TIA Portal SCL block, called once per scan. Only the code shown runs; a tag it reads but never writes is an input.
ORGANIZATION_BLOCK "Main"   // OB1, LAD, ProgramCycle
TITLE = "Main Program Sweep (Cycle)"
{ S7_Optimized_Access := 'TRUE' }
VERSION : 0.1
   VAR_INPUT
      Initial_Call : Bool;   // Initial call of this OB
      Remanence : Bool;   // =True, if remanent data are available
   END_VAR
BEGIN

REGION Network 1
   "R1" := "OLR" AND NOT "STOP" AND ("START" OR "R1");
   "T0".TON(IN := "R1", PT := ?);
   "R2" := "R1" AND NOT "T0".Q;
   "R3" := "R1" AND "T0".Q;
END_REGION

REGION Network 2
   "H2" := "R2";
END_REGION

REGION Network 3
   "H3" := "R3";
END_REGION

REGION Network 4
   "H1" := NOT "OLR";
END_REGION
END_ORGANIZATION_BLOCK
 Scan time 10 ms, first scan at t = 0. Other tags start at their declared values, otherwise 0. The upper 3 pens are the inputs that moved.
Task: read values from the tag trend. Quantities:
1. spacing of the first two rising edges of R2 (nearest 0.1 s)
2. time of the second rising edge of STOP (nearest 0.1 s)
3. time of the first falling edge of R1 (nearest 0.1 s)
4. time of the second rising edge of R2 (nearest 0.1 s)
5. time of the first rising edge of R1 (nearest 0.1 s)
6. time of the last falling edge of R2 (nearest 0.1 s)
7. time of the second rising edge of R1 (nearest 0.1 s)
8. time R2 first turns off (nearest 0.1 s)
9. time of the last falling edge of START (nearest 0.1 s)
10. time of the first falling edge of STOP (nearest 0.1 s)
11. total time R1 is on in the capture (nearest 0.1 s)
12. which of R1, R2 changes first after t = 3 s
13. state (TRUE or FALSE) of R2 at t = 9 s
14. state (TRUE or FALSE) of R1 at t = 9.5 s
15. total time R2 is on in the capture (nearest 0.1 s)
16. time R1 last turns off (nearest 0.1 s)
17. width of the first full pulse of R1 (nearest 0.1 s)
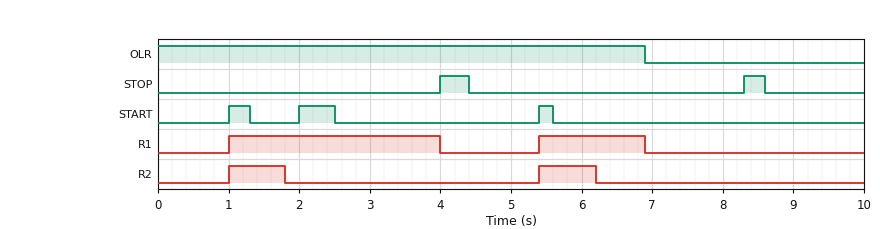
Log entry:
4.4 s
8.3 s
4.0 s
5.4 s
1.0 s
6.2 s
5.4 s
1.8 s
5.6 s
4.4 s
4.5 s
R1
FALSE
FALSE
1.6 s
6.9 s
3.0 s
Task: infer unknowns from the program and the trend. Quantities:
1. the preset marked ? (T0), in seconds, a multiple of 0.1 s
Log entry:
0.8 s
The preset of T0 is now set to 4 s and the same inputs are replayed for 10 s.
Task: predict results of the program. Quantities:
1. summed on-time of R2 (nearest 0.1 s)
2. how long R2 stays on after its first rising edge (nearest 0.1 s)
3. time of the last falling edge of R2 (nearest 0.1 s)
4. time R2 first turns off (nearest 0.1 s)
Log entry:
4.5 s
3.0 s
6.9 s
4.0 s
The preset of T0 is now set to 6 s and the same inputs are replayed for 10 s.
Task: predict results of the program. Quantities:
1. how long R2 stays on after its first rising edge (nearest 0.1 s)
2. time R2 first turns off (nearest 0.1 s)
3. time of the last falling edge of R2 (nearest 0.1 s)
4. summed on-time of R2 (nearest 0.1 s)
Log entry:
3.0 s
4.0 s
6.9 s
4.5 s
